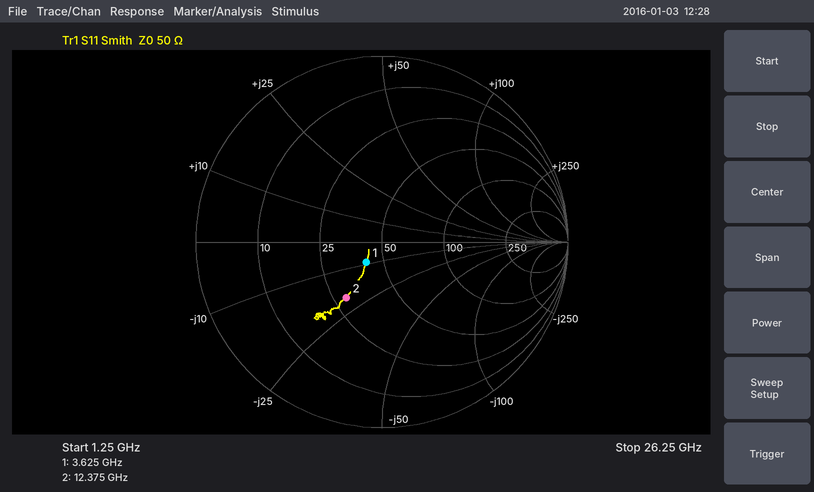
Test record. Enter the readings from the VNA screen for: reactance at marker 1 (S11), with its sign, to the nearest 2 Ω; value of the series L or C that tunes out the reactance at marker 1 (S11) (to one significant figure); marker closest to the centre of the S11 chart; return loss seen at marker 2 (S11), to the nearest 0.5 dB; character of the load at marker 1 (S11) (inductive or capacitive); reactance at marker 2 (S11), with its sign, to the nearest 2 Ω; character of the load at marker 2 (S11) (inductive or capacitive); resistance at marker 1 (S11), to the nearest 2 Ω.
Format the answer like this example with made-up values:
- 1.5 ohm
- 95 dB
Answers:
- -10 Ω
- 400 pH
- marker 1
- 9.0 dB
- capacitive
- -20 Ω
- capacitive
- 42 Ω
